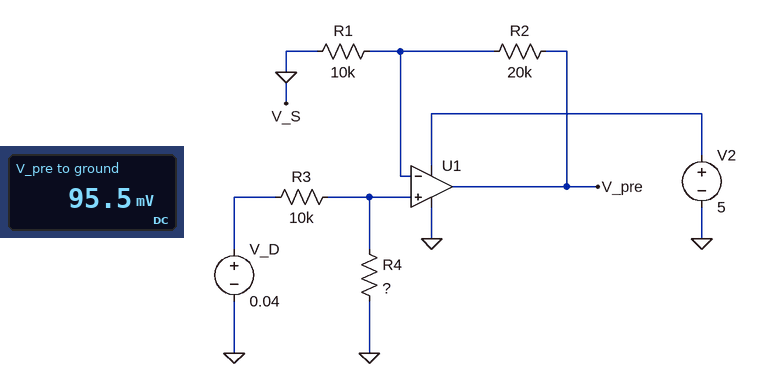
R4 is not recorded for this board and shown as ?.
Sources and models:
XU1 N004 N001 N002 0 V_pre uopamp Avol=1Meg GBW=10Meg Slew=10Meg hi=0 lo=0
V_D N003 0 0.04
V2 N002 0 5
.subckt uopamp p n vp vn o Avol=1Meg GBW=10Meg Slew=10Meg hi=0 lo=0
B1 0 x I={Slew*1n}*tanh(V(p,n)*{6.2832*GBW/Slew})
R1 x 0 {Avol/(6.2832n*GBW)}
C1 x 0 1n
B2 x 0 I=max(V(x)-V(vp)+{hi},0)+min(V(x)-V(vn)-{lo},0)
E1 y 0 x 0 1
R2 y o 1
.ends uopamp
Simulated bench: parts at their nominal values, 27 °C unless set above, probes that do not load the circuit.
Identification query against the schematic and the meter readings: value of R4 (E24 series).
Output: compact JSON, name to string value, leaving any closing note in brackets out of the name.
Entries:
{"value of R4": "39 kΩ"}
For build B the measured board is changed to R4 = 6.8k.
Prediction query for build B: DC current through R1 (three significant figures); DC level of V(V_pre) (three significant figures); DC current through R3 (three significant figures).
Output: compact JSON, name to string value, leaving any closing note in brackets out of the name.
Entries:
{"DC current through R1": "1.62 µA", "DC level of V(V_pre)": "48.6 mV", "DC current through R3": "2.38 µA"}
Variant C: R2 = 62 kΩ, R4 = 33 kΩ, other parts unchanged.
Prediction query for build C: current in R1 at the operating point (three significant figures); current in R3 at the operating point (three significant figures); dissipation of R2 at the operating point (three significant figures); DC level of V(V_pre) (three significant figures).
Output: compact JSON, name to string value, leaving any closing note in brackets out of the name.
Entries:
{"current in R1 at the operating point": "3.07 µA", "current in R3 at the operating point": "930 nA", "dissipation of R2 at the operating point": "584 nW", "DC level of V(V_pre)": "221 mV"}
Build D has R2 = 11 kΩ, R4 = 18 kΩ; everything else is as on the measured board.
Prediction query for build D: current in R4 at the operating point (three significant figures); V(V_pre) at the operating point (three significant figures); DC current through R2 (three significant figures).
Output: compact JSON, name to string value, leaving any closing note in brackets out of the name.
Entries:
{"current in R4 at the operating point": "1.43 µA", "V(V_pre) at the operating point": "54.0 mV", "DC current through R2": "2.57 µA"}
